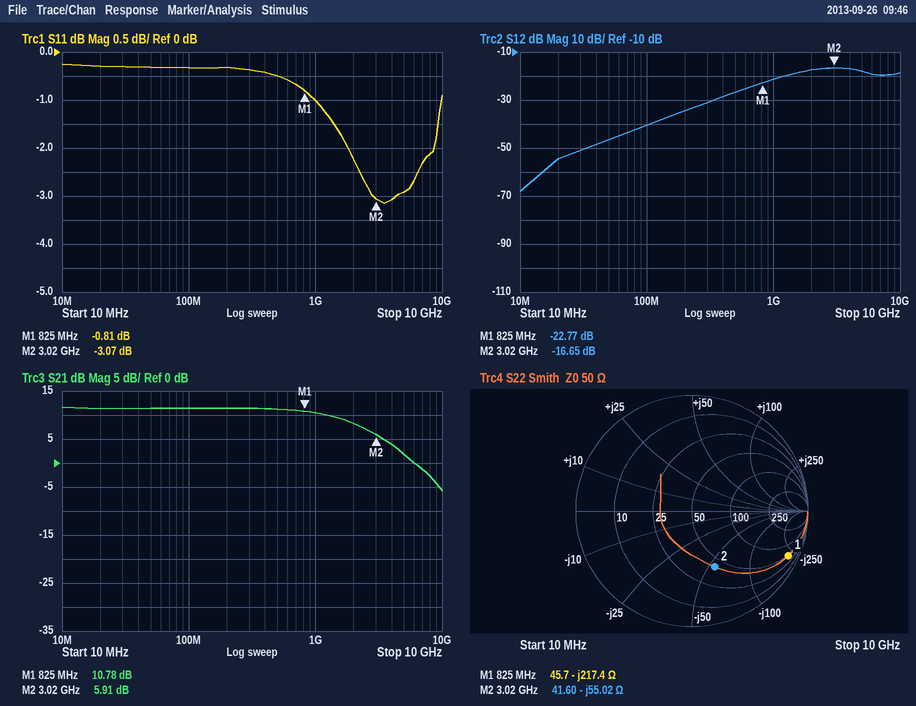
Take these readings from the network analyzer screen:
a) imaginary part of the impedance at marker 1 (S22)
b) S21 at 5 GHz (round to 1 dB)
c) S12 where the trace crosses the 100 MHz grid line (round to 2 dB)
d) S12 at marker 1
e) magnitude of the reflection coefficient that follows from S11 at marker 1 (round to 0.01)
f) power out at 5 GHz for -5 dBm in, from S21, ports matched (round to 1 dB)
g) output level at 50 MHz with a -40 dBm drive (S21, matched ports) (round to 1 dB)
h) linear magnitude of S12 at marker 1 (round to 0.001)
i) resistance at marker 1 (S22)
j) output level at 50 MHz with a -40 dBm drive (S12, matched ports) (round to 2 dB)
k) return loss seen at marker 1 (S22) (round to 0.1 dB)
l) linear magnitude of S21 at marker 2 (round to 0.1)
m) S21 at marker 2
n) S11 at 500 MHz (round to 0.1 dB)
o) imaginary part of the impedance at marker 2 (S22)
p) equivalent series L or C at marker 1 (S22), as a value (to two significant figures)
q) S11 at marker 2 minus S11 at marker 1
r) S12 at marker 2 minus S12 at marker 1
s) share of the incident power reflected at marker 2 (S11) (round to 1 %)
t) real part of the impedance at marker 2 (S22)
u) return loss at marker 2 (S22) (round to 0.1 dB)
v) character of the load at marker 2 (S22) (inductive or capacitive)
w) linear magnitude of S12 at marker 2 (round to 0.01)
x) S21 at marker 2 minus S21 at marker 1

-217.4 Ω
2 dB
-40 dB
-22.77 dB
0.91
-3 dBm
-29 dBm
0.073
45.7 Ω
-86 dBm
0.8 dB
2.0
5.91 dB
-0.5 dB
-55.02 Ω
890 fF
-2.26 dB
6.12 dB
49 %
41.60 Ω
5.7 dB
capacitive
0.15
-4.87 dB
